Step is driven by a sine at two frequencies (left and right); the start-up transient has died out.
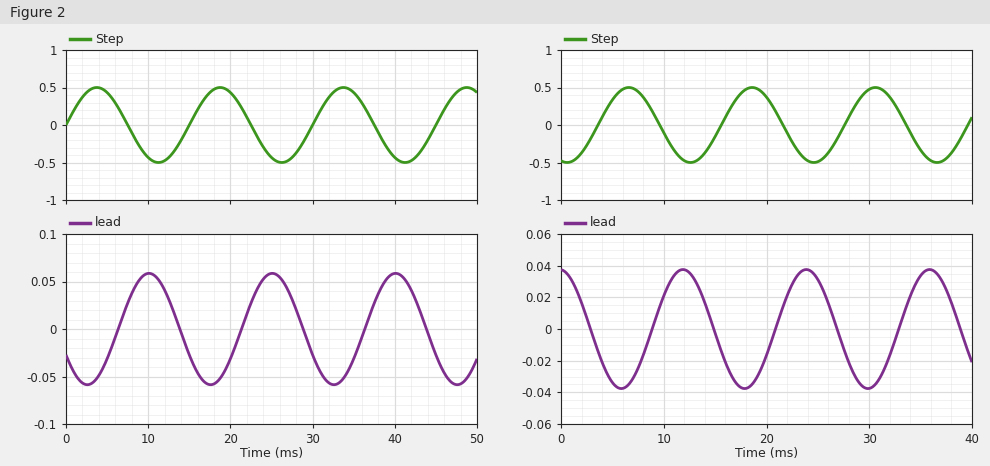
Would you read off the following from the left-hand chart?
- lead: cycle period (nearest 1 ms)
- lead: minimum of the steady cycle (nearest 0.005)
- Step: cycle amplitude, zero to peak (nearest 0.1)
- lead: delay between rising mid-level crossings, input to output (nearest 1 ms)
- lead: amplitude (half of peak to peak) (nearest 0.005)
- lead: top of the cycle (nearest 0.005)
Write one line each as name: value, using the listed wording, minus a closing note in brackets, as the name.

lead: cycle period: 15 ms
lead: minimum of the steady cycle: -0.060
Step: cycle amplitude, zero to peak: 0.5
lead: delay between rising mid-level crossings, input to output: 6 ms
lead: amplitude (half of peak to peak): 0.060
lead: top of the cycle: 0.060
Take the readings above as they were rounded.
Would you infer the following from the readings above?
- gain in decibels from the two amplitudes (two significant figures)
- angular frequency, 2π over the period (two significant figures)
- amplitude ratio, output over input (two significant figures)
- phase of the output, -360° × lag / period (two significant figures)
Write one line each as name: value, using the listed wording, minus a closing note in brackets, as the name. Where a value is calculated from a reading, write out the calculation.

gain in decibels from the two amplitudes: 20 log10(0.06 / 0.5) = -18 dB
angular frequency, 2π over the period: 2π / 15 = 0.42 rad/ms
amplitude ratio, output over input: 0.06 / 0.5 = 0.12
phase of the output, -360° × lag / period: -360 × 6 / 15 = -140°
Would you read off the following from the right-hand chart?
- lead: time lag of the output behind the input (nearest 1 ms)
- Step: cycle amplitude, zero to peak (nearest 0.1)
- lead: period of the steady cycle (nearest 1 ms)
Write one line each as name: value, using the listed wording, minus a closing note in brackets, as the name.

lead: time lag of the output behind the input: 5 ms
Step: cycle amplitude, zero to peak: 0.5
lead: period of the steady cycle: 12 ms
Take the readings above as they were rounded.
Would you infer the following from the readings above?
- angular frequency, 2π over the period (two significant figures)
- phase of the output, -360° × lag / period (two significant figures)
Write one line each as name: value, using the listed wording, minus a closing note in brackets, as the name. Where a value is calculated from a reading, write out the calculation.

angular frequency, 2π over the period: 2π / 12 = 0.52 rad/ms
phase of the output, -360° × lag / period: -360 × 5 / 12 = -150°
